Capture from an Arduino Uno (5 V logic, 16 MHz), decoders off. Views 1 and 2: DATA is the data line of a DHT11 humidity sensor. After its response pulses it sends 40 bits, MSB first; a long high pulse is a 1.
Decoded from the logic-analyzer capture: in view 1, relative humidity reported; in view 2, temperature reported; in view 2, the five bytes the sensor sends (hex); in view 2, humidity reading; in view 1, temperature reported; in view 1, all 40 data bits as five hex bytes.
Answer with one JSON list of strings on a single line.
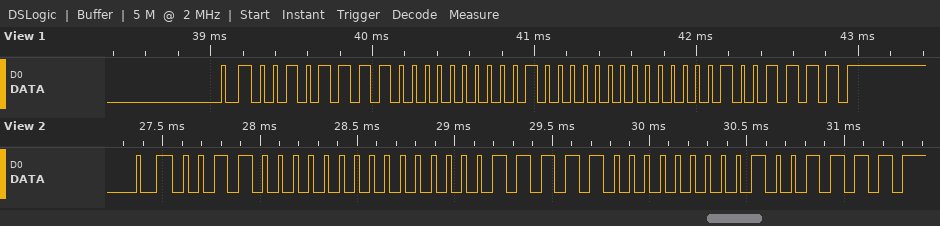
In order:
["47 %", "31.0 °C", "30 00 1F 00 4F", "48 %", "32.0 °C", "2F 00 20 00 4F"]
